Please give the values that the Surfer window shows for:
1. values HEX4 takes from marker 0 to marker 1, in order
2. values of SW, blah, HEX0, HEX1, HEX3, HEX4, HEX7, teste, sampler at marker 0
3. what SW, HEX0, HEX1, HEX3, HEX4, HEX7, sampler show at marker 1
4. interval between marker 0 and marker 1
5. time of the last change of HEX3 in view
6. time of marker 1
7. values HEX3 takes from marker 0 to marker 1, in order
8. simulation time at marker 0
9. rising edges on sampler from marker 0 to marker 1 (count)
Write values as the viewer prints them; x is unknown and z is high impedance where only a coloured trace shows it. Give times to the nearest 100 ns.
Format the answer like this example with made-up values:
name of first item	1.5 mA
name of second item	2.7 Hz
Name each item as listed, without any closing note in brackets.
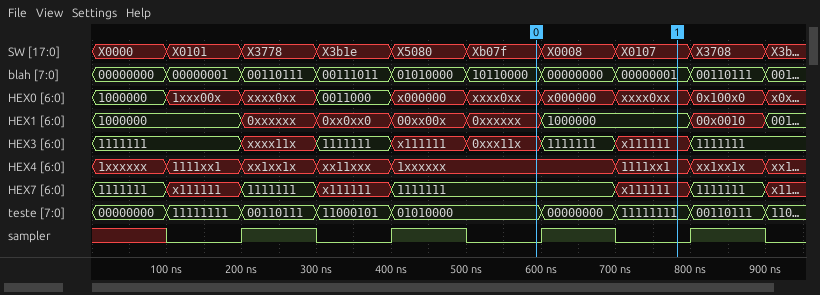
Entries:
values HEX4 takes from marker 0 to marker 1, in order	1xxxxxx, 1111xx1
values of SW, blah, HEX0, HEX1, HEX3, HEX4, HEX7, teste, sampler at marker 0	SW=Xb07f, blah=10110000, HEX0=xxxx0xx, HEX1=0xxxxxx, HEX3=0xxx11x, HEX4=1xxxxxx, HEX7=1111111, teste=01010000, sampler=0
what SW, HEX0, HEX1, HEX3, HEX4, HEX7, sampler show at marker 1	SW=X0107, HEX0=xxxx0xx, HEX1=1000000, HEX3=x111111, HEX4=1111xx1, HEX7=x111111, sampler=0
interval between marker 0 and marker 1	200 ns
time of the last change of HEX3 in view	800 ns
time of marker 1	800 ns
values HEX3 takes from marker 0 to marker 1, in order	0xxx11x, 1111111, x111111
simulation time at marker 0	600 ns
rising edges on sampler from marker 0 to marker 1	1
